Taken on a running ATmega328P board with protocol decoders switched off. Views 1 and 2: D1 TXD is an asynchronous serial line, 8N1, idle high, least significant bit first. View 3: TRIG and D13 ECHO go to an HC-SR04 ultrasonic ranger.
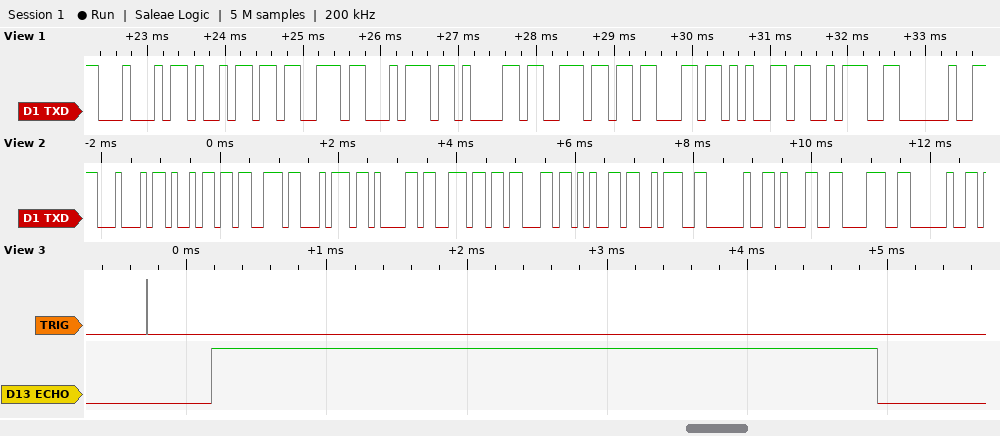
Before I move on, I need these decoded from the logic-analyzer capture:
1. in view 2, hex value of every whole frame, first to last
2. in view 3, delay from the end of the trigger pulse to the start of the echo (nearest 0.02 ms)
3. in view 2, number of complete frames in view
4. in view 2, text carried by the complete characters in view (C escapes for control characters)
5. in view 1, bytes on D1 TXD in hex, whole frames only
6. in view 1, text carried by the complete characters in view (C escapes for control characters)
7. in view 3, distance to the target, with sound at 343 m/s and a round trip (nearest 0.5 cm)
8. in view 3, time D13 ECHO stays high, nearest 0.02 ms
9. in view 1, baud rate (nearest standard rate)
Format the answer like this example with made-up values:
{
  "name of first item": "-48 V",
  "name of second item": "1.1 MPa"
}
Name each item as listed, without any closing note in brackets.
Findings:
{
  "in view 2, hex value of every whole frame, first to last": "44 69 73 74 61 6E 63 65 3A 20 31 38 20",
  "in view 3, delay from the end of the trigger pulse to the start of the echo": "0.46 ms",
  "in view 2, number of complete frames in view": "13",
  "in view 2, text carried by the complete characters in view": "\"Distance: 18 \"",
  "in view 1, bytes on D1 TXD in hex, whole frames only": "0x44 0x69 0x73 0x74 0x61 0x6E 0x63 0x65 0x3A 0x20",
  "in view 1, text carried by the complete characters in view": "\"Distance: \"",
  "in view 3, distance to the target, with sound at 343 m/s and a round trip": "81.5 cm",
  "in view 3, time D13 ECHO stays high, nearest 0.02 ms": "4.76 ms",
  "in view 1, baud rate": "9600 baud"
}
